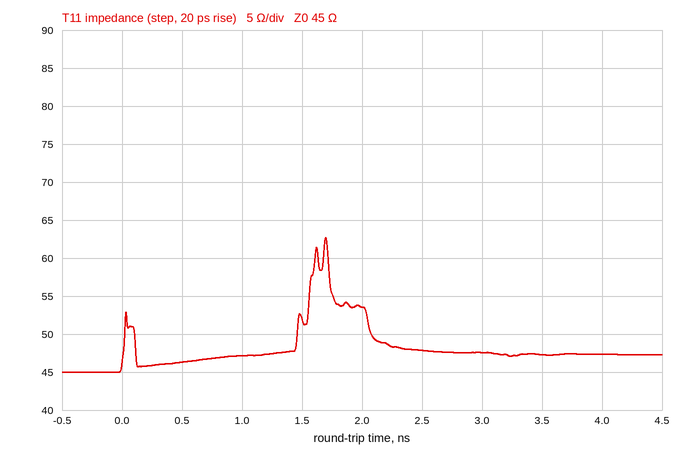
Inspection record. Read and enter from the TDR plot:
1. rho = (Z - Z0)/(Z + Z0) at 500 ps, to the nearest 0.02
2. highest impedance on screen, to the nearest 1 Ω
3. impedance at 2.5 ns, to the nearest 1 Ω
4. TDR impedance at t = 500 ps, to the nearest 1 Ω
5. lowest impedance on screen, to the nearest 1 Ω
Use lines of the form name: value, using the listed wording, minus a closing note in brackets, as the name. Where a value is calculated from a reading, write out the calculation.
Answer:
rho = (Z - Z0)/(Z + Z0) at 500 ps, to the nearest 0.02: (46 − 45)/(46 + 45) ≈ +0.0110, so +0.02 to the nearest 0.02
highest impedance on screen, to the nearest 1 Ω: 63 Ω
impedance at 2.5 ns, to the nearest 1 Ω: 48 Ω
TDR impedance at t = 500 ps, to the nearest 1 Ω: 46 Ω
lowest impedance on screen, to the nearest 1 Ω: 45 Ω
